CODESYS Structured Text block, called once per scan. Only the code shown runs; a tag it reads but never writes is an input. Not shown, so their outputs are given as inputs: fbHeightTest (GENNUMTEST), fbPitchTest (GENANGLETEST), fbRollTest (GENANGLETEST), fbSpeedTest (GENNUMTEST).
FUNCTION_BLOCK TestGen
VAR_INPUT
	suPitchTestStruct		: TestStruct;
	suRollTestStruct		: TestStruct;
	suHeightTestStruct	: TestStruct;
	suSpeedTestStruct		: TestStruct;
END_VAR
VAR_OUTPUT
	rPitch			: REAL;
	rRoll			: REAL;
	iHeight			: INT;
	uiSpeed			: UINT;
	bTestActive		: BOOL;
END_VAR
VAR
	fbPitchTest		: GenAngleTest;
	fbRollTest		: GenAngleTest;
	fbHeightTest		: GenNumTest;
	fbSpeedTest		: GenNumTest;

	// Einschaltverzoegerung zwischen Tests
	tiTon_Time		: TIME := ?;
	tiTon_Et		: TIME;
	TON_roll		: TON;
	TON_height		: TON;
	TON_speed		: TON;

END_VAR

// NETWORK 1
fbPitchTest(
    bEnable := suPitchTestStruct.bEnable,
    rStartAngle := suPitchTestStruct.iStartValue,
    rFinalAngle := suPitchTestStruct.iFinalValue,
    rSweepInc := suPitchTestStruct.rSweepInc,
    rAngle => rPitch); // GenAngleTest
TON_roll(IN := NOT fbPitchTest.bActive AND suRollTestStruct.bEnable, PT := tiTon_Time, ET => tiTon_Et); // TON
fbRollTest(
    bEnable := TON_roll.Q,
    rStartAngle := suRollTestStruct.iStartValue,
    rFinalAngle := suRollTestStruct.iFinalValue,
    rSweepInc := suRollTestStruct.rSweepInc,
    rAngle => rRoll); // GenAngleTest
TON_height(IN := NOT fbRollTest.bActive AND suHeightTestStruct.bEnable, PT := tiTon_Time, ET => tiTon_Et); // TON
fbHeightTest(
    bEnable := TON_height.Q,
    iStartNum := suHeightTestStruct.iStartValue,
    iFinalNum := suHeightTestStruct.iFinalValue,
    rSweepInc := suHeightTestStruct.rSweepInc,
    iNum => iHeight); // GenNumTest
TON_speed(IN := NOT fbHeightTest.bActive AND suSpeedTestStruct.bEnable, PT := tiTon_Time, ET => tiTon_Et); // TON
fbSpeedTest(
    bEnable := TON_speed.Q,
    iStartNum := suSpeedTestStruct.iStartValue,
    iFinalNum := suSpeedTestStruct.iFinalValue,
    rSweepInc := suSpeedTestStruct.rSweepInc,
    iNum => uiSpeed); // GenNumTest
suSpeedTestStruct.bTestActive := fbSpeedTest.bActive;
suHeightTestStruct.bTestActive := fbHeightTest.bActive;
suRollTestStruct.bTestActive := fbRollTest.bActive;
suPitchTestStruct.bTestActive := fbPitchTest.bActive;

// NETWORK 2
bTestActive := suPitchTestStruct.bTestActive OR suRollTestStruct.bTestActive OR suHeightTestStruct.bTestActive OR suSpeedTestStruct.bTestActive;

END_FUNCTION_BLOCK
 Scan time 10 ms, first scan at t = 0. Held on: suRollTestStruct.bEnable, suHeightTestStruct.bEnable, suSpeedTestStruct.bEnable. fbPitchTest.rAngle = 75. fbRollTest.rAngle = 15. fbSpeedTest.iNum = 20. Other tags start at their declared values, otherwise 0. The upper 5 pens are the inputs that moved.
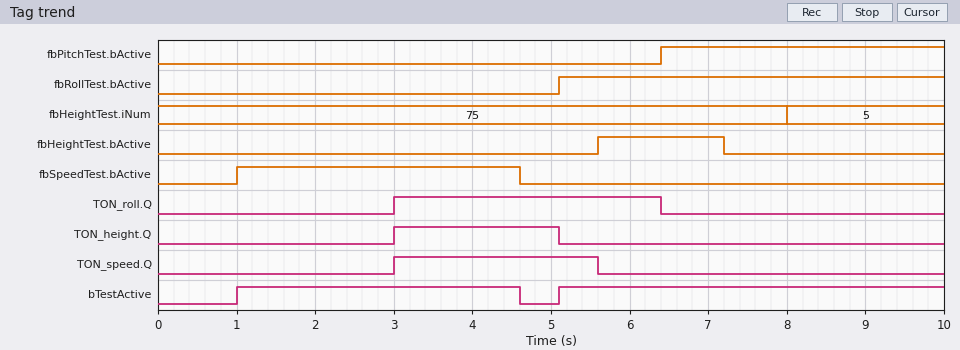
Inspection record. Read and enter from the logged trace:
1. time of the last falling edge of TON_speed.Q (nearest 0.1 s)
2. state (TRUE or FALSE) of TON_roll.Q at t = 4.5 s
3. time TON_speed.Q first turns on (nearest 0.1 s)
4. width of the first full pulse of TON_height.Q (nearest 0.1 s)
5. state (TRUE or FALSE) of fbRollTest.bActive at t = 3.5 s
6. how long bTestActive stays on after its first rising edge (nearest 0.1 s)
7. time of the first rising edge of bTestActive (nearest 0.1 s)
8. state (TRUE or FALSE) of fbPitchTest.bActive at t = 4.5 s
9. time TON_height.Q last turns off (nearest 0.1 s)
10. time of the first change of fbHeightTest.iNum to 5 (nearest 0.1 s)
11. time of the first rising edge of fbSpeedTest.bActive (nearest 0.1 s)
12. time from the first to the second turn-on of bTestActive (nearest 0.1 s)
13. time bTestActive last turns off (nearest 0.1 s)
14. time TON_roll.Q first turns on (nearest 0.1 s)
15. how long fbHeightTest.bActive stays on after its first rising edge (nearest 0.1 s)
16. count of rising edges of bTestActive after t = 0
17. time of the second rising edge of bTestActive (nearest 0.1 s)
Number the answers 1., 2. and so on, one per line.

1. 5.6 s
2. TRUE
3. 3.0 s
4. 2.1 s
5. FALSE
6. 3.6 s
7. 1.0 s
8. FALSE
9. 5.1 s
10. 8.0 s
11. 1.0 s
12. 4.1 s
13. 4.6 s
14. 3.0 s
15. 1.6 s
16. 2
17. 5.1 s
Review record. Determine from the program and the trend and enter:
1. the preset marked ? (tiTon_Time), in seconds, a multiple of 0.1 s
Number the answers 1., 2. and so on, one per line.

1. 3.0 s
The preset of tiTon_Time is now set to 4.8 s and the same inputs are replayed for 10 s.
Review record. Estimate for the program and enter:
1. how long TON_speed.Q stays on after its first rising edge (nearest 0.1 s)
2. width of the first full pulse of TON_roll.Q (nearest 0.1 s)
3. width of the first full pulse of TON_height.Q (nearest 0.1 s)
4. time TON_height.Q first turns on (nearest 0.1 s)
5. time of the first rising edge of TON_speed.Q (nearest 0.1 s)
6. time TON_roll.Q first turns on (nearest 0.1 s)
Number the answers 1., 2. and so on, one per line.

1. 0.8 s
2. 1.6 s
3. 0.3 s
4. 4.8 s
5. 4.8 s
6. 4.8 s
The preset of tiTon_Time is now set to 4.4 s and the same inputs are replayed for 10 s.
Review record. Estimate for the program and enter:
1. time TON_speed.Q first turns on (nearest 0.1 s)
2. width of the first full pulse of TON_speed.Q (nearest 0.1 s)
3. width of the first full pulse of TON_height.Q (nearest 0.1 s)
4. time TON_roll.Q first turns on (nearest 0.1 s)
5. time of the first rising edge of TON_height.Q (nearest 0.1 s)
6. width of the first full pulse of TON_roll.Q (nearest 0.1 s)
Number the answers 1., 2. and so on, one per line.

1. 4.4 s
2. 1.2 s
3. 0.7 s
4. 4.4 s
5. 4.4 s
6. 2.0 s
